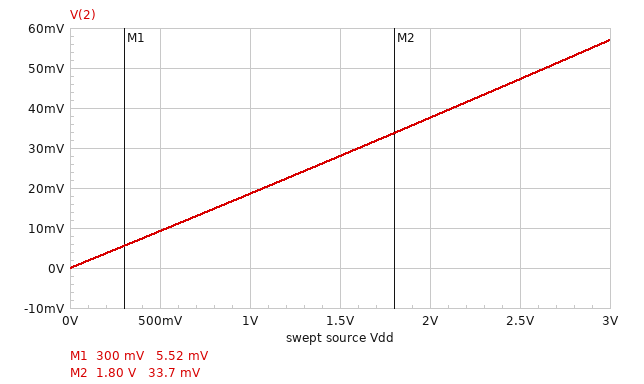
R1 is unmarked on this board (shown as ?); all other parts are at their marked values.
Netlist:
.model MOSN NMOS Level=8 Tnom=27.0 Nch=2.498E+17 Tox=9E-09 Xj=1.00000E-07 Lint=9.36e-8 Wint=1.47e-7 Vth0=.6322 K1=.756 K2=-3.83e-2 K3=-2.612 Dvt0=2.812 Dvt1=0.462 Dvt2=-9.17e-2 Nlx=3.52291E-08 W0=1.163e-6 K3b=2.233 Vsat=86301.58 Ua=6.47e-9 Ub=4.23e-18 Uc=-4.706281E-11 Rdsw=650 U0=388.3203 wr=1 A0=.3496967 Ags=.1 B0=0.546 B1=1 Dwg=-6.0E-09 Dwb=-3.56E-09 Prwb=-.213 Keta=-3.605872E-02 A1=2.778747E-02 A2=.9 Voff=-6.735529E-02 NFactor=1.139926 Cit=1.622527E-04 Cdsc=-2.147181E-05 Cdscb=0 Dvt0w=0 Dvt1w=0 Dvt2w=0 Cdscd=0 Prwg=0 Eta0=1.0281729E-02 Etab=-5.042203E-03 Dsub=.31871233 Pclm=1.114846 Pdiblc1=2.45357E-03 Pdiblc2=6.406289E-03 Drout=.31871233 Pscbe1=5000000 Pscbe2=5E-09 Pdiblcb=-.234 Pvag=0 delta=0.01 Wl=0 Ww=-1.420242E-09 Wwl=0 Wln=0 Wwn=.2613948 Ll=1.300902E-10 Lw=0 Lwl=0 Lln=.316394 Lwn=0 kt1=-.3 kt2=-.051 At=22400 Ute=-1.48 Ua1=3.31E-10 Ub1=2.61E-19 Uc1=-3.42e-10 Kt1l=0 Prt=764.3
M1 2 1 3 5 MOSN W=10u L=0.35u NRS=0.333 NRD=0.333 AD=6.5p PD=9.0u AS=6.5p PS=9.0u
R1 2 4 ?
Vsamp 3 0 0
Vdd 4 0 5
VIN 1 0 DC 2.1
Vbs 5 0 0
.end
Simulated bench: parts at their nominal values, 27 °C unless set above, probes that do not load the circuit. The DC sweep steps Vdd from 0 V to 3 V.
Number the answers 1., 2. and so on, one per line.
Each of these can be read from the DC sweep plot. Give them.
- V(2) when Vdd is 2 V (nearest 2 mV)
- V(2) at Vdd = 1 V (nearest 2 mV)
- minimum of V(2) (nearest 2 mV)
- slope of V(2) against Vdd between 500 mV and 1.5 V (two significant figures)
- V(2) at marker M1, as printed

1. 38 mV
2. 18 mV
3. 0 V
4. 0.019 V/V
5. 5.52 mV
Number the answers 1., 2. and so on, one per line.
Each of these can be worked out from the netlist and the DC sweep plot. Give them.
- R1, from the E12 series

1. 12 kΩ
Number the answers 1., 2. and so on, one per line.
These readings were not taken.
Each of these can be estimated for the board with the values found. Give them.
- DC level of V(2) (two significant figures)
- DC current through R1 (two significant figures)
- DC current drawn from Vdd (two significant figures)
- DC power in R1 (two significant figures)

1. 97 mV
2. 410 µA
3. 410 µA
4. 2.0 mW
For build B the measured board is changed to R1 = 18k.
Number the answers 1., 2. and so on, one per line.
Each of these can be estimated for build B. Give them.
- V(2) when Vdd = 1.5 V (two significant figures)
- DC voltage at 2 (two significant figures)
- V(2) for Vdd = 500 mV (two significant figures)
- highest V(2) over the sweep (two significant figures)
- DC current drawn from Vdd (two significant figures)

1. 19 mV
2. 64 mV
3. 6.2 mV
4. 38 mV
5. 270 µA
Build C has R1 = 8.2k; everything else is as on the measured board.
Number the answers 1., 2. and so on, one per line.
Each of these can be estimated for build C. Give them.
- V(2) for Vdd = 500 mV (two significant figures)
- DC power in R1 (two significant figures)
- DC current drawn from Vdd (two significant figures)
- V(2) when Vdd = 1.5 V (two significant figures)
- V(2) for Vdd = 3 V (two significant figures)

1. 13 mV
2. 2.9 mW
3. 590 µA
4. 41 mV
5. 84 mV
